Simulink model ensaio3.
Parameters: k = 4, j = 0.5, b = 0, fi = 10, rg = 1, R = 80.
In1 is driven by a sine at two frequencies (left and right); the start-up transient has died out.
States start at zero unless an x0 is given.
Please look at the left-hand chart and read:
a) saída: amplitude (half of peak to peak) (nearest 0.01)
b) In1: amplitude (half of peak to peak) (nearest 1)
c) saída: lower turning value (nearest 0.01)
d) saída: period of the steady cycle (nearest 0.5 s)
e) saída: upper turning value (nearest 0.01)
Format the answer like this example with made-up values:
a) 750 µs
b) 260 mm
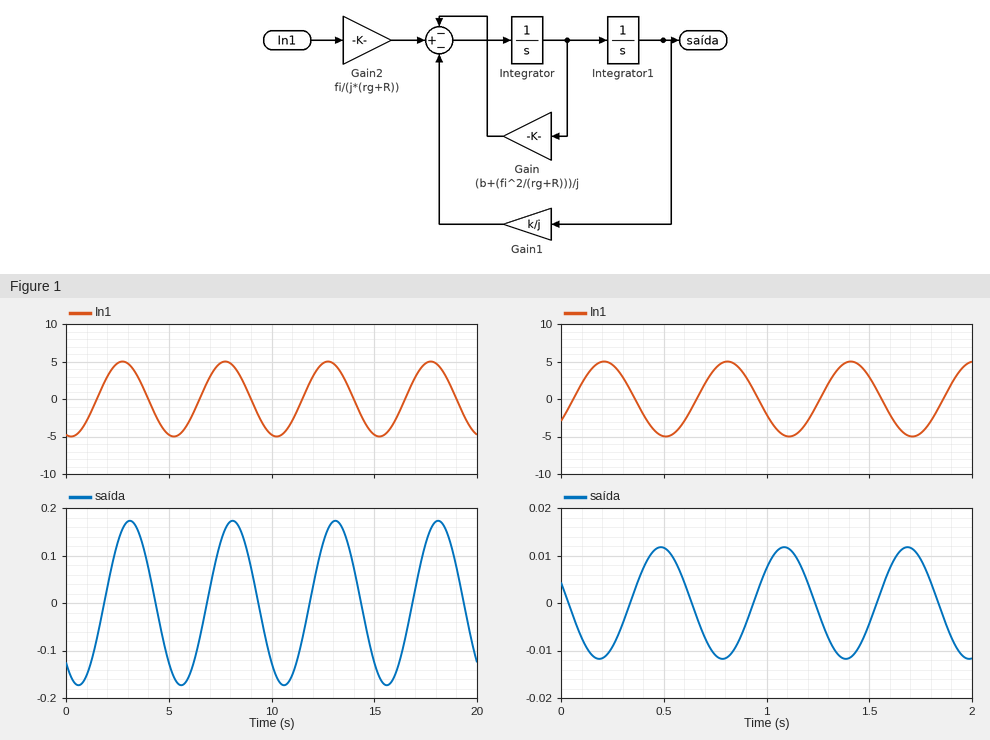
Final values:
a) 0.17
b) 5
c) -0.17
d) 5.0 s
e) 0.17
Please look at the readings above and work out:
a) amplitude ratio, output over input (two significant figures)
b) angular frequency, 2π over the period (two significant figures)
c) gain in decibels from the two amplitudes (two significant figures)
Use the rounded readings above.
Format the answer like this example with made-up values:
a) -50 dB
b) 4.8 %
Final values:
a) 0.034
b) 1.3 rad/s
c) -29 dB
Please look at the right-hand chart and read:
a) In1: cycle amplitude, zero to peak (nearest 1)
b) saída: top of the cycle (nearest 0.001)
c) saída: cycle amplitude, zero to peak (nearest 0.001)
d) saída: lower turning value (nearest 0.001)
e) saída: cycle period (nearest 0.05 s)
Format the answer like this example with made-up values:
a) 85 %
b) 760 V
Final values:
a) 5
b) 0.012
c) 0.012
d) -0.012
e) 0.60 s
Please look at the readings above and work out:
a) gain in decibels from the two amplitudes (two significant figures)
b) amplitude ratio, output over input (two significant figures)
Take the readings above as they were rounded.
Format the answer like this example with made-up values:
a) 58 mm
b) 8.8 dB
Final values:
a) -52 dB
b) 0.0024
